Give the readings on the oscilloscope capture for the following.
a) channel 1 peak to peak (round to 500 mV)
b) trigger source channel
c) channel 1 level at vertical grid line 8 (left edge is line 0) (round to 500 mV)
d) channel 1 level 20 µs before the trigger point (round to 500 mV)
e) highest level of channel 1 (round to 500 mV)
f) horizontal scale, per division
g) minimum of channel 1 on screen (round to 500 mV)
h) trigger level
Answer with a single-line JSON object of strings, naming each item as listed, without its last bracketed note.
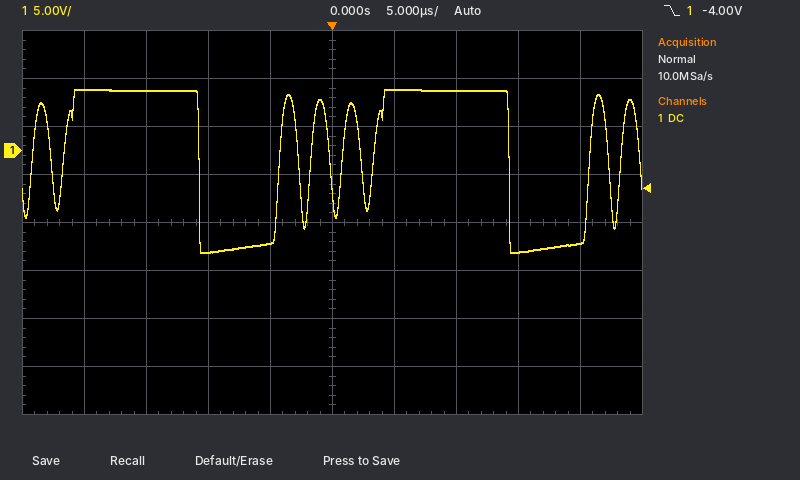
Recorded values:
{"channel 1 peak to peak": "17.0 V", "trigger source channel": "channel 1", "channel 1 level at vertical grid line 8 (left edge is line 0)": "-10.5 V", "channel 1 level 20 µs before the trigger point": "6.5 V", "highest level of channel 1": "6.5 V", "horizontal scale, per division": "5 µs", "minimum of channel 1 on screen": "-10.5 V", "trigger level": "-4.00 V"}
